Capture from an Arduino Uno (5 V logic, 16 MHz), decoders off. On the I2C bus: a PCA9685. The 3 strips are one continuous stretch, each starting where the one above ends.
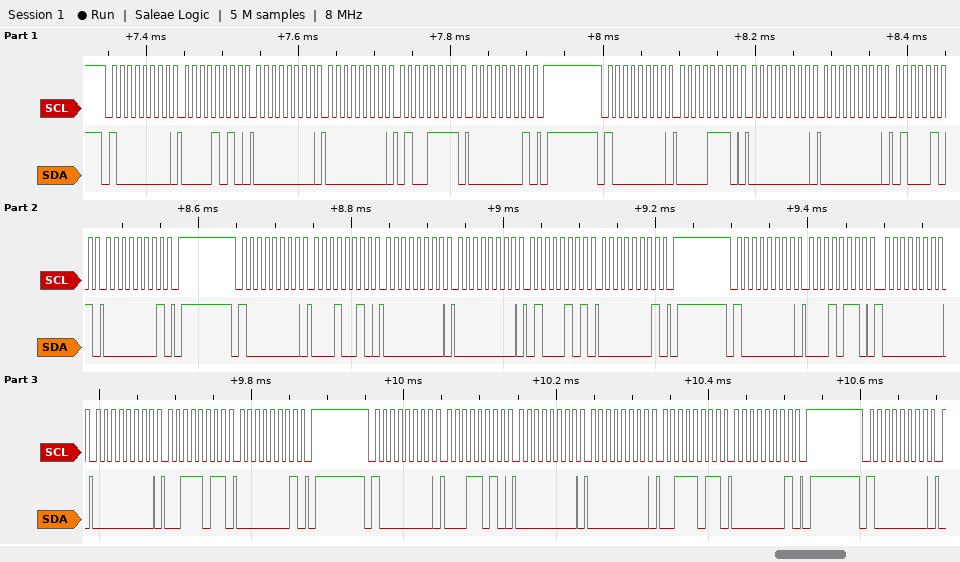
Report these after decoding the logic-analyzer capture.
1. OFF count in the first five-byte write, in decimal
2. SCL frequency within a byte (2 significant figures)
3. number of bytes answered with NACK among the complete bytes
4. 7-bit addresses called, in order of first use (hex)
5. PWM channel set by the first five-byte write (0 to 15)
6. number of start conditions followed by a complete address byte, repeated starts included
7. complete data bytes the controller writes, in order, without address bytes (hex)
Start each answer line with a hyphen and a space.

- 335
- 100 kHz
- 0
- 0x40
- 1
- 6
- 0A 00 00 4F 01 0E 00 00 45 01 12 00 00 45 01 16 00 00 3B 01 1A 00 00 3B 01
